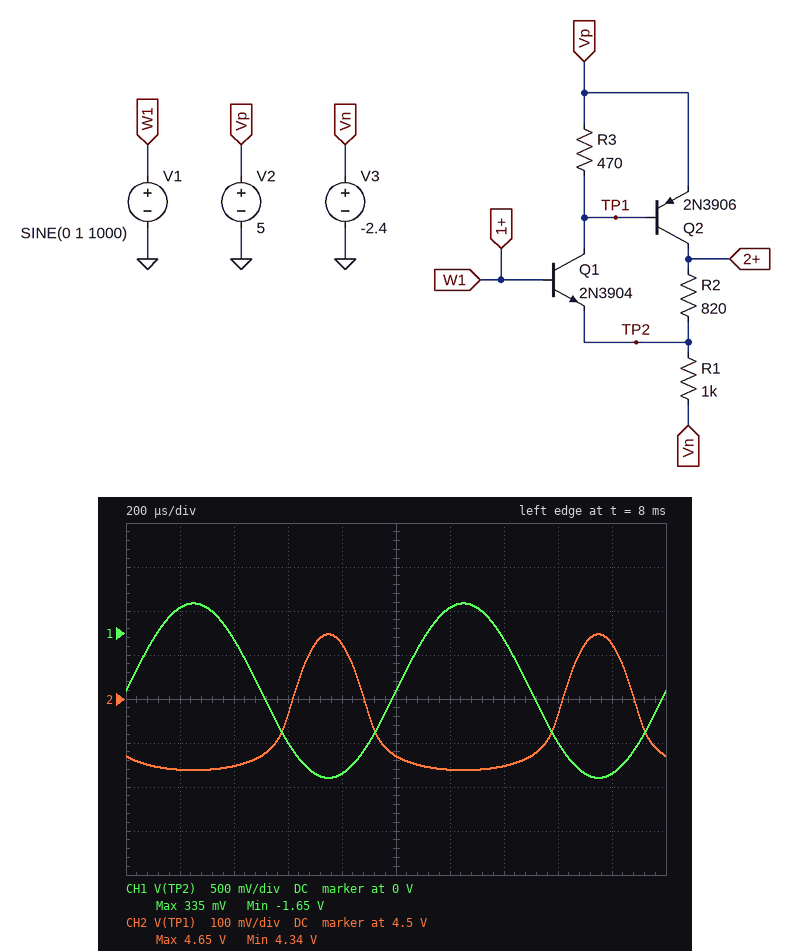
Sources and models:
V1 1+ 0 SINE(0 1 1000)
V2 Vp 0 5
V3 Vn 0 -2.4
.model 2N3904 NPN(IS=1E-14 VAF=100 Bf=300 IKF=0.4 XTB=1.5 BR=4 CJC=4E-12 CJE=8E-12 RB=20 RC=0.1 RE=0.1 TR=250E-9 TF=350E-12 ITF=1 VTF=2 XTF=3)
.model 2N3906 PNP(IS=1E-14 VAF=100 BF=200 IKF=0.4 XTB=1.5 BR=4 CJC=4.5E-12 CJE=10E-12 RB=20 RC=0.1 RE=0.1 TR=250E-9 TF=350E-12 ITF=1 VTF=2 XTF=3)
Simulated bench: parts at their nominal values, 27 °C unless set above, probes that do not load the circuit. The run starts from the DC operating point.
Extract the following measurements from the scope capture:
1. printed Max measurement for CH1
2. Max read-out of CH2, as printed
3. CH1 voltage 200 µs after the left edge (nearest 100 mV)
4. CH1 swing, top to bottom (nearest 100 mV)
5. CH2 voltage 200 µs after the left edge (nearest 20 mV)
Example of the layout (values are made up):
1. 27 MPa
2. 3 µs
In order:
1. 335 mV
2. 4.65 V
3. 300 mV
4. 2.0 V
5. 4.34 V
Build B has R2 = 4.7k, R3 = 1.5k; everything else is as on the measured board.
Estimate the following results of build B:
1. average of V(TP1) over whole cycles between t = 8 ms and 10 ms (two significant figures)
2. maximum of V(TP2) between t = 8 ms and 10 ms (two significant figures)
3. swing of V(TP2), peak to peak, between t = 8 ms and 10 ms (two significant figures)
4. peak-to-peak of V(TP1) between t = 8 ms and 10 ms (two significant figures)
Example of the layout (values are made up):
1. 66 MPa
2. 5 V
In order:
1. 4.3 V
2. 330 mV
3. 2.0 V
4. 100 mV
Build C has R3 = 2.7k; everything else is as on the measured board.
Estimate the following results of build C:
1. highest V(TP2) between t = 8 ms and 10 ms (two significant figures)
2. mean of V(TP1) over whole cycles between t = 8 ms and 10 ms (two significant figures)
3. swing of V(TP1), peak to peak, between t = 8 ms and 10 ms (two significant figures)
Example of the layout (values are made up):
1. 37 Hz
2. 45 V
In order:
1. 380 mV
2. 4.3 V
3. 41 mV
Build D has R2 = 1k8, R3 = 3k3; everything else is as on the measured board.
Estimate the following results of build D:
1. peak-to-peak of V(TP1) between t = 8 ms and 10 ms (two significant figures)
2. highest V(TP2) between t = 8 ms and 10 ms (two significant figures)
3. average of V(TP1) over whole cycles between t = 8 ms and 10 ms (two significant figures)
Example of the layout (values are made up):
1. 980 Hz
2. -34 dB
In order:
1. 42 mV
2. 380 mV
3. 4.3 V
